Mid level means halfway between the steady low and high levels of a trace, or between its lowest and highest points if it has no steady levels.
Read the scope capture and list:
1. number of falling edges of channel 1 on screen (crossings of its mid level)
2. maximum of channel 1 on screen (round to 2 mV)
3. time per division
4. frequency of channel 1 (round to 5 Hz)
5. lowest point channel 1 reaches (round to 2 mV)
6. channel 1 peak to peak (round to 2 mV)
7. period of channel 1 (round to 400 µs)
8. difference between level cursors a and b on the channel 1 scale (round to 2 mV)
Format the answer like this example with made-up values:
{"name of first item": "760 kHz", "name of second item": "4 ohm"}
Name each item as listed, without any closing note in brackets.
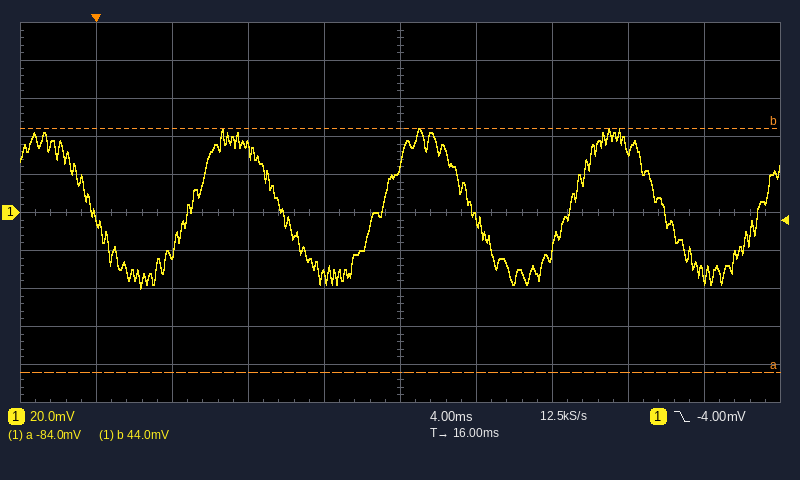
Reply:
{"number of falling edges of channel 1 on screen": "4", "maximum of channel 1 on screen": "44 mV", "time per division": "4 ms", "frequency of channel 1": "100 Hz", "lowest point channel 1 reaches": "-40 mV", "channel 1 peak to peak": "84 mV", "period of channel 1": "10.0 ms", "difference between level cursors a and b on the channel 1 scale": "128 mV"}
